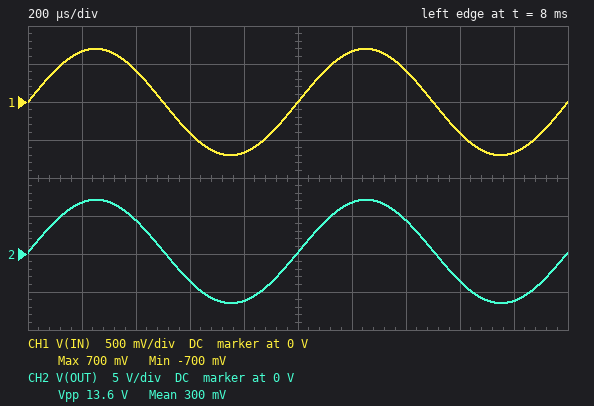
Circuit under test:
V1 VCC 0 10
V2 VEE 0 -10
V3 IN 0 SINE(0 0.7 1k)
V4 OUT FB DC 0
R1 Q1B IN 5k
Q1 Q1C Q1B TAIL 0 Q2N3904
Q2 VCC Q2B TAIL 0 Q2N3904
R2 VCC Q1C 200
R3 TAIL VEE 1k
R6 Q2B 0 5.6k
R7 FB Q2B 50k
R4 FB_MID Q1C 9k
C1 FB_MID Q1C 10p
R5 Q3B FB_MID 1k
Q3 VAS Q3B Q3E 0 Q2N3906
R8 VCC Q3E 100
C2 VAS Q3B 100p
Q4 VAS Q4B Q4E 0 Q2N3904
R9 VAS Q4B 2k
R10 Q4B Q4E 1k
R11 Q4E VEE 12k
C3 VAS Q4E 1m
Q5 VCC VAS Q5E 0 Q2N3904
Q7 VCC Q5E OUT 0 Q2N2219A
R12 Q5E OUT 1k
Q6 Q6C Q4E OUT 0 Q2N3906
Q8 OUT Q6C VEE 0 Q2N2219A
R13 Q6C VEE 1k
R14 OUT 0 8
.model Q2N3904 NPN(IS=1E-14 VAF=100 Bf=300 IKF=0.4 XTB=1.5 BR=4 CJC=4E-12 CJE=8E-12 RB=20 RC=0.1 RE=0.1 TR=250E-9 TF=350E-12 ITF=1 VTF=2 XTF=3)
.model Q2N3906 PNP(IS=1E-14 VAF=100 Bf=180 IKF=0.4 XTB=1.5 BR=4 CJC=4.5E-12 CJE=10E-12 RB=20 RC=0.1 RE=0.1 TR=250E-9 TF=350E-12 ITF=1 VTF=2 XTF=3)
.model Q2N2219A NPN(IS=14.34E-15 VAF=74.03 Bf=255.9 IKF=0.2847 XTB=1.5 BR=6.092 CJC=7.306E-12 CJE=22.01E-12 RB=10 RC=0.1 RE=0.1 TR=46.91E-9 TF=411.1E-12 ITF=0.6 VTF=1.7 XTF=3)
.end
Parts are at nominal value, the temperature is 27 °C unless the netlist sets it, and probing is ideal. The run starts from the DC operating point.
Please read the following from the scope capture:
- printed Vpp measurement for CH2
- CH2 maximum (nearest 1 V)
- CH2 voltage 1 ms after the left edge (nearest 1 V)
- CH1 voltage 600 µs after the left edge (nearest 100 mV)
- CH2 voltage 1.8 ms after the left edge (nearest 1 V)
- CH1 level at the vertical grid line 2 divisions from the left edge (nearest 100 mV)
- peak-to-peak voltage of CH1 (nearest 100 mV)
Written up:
13.6 V
7 V
0 V
-400 mV
-6 V
400 mV
1.4 V
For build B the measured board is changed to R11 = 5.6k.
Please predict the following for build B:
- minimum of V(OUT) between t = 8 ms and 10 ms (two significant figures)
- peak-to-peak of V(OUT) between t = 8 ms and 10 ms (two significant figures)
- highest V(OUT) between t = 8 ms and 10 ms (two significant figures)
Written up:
-6.6 V
13 V
6.6 V
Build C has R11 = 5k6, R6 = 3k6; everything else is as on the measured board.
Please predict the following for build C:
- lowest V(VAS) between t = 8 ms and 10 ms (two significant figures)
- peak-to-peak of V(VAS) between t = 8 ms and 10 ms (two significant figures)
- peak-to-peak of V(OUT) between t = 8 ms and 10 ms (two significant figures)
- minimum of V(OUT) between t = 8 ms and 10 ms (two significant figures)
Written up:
-7.4 V
17 V
16 V
-8.6 V
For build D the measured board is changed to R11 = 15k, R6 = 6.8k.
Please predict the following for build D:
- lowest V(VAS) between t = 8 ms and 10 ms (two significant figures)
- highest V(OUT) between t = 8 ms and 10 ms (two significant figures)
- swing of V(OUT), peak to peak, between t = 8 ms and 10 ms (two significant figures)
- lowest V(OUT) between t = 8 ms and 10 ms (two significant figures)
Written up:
-4.3 V
6.3 V
12 V
-5.3 V
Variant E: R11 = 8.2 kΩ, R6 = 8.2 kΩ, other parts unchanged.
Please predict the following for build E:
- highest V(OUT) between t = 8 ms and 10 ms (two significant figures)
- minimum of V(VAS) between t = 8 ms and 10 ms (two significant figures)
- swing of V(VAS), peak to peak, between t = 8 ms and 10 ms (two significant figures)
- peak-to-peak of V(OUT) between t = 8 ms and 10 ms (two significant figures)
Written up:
5.2 V
-3.3 V
10 V
9.8 V
